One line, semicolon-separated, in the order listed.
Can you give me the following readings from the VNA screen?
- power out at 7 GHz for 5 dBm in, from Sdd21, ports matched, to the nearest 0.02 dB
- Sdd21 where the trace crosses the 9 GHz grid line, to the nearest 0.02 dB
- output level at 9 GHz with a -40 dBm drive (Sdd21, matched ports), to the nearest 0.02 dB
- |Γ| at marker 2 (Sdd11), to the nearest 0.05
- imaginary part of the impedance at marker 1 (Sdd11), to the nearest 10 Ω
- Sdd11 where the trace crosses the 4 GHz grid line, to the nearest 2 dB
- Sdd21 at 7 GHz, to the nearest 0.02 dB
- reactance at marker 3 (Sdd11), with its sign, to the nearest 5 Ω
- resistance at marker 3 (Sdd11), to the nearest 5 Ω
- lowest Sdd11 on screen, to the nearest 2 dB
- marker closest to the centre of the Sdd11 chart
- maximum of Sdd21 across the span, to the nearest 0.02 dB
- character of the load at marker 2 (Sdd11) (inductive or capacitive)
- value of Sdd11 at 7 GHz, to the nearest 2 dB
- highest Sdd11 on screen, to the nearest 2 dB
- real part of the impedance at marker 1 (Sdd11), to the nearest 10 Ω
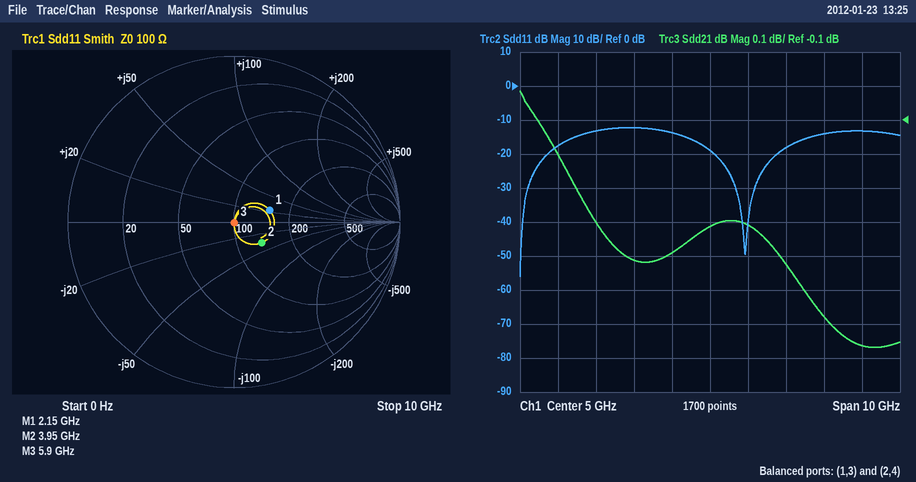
4.48 dBm; -0.76 dB; -40.76 dBm; 0.20; +20 Ω; -14 dB; -0.52 dB; 0 Ω; 100 Ω; -56 dB; marker 3; -0.02 dB; capacitive; -18 dB; -12 dB; 150 Ω
